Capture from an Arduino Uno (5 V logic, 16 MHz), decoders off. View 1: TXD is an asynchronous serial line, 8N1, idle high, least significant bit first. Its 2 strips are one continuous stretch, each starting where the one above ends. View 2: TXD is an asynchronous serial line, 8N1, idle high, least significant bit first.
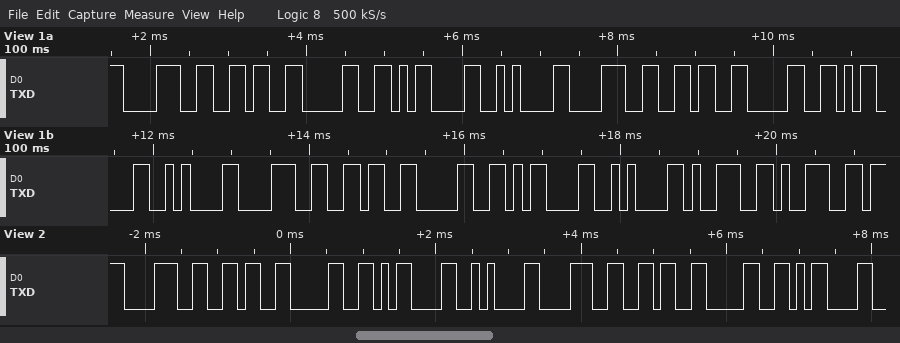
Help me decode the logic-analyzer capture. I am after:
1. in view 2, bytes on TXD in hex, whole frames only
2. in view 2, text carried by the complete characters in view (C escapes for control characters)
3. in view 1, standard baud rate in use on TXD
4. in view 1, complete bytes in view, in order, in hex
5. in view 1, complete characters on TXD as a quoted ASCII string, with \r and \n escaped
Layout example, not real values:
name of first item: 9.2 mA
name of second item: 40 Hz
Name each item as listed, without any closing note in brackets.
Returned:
in view 2, bytes on TXD in hex, whole frames only: 38 36 30 0D 0A 38 36 30 0D
in view 2, text carried by the complete characters in view: "860\r\n860\r"
in view 1, standard baud rate in use on TXD: 9600 baud
in view 1, complete bytes in view, in order, in hex: 38 36 30 0D 0A 38 36 30 0D 0A 38 36 30 0D 0A 39 39
in view 1, complete characters on TXD as a quoted ASCII string, with \r and \n escaped: "860\r\n860\r\n860\r\n99"
